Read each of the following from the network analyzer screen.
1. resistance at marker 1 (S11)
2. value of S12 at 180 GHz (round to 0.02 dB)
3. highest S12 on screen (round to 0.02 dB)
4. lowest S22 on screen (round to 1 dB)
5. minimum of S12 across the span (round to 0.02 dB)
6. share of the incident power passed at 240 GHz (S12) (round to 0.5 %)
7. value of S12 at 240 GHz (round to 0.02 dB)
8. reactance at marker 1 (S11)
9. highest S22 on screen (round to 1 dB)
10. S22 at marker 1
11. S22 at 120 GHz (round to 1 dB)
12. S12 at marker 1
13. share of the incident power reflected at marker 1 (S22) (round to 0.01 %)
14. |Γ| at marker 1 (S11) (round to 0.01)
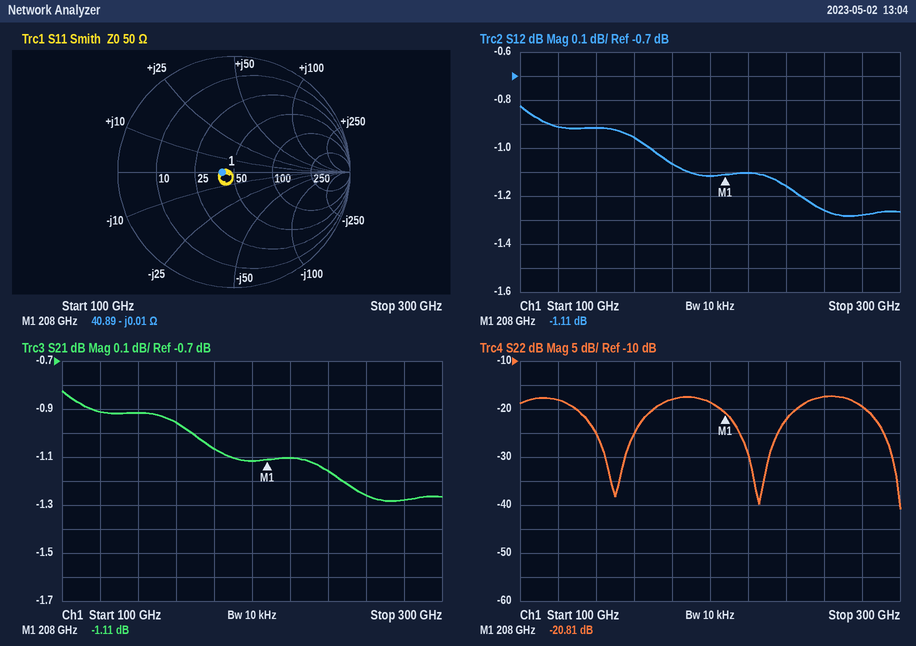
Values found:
40.89 Ω
-1.06 dB
-0.82 dB
-41 dB
-1.28 dB
76.5 %
-1.16 dB
-0.01 Ω
-17 dB
-20.81 dB
-18 dB
-1.11 dB
0.83 %
0.10
